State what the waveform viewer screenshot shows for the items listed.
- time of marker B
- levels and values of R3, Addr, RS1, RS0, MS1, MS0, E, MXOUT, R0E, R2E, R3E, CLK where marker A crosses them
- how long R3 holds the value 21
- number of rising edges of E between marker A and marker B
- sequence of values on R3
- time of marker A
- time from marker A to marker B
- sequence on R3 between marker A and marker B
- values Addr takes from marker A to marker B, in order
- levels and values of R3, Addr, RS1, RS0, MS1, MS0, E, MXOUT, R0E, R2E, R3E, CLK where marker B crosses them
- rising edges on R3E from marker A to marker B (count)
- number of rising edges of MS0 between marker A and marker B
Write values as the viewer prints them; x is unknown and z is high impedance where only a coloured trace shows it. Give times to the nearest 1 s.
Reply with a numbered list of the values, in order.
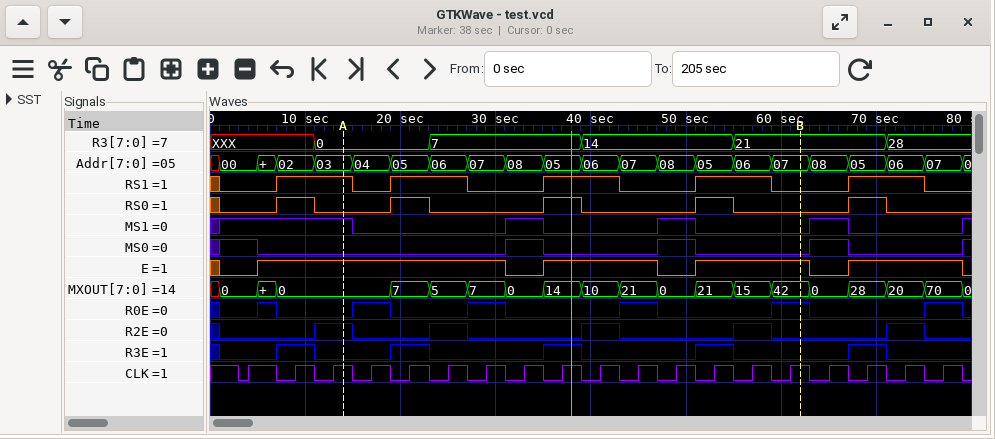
1. 62 s
2. R3=0, Addr=03, RS1=1, RS0=0, MS1=1, MS0=0, E=1, MXOUT=0, R0E=0, R2E=1, R3E=0, CLK=1
3. 16 s
4. 2
5. XXX, 0, 7, 14, 21, 28
6. 14 s
7. 48 s
8. 0, 7, 14, 21
9. 03, 04, 05, 06, 07, 08, 05, 06, 07, 08, 05, 06, 07
10. R3=21, Addr=07, RS1=0, RS0=0, MS1=0, MS0=0, E=1, MXOUT=42, R0E=1, R2E=0, R3E=0, CLK=1
11. 3
12. 2
